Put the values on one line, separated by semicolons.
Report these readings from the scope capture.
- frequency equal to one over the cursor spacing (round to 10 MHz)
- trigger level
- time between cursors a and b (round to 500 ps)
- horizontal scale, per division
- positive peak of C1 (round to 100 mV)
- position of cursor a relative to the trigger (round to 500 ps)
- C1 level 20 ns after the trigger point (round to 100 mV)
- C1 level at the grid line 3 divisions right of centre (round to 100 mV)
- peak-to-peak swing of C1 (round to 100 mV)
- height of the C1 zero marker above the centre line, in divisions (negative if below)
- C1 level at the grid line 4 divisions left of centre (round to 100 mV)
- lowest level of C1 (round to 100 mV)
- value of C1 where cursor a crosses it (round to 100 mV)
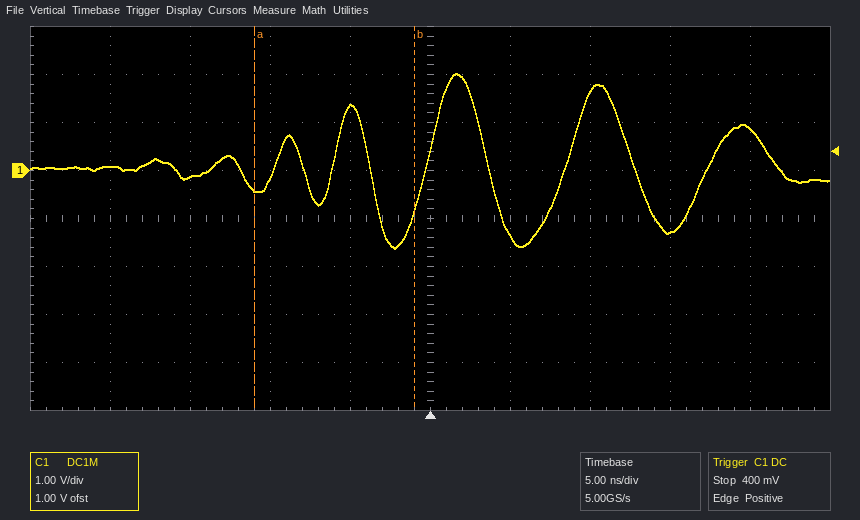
100 MHz; 400 mV; 10.0 ns; 5 ns; 2.0 V; -11.0 ns; 900 mV; -1.3 V; 3.6 V; +1.0 div; 100 mV; -1.6 V; -400 mV
